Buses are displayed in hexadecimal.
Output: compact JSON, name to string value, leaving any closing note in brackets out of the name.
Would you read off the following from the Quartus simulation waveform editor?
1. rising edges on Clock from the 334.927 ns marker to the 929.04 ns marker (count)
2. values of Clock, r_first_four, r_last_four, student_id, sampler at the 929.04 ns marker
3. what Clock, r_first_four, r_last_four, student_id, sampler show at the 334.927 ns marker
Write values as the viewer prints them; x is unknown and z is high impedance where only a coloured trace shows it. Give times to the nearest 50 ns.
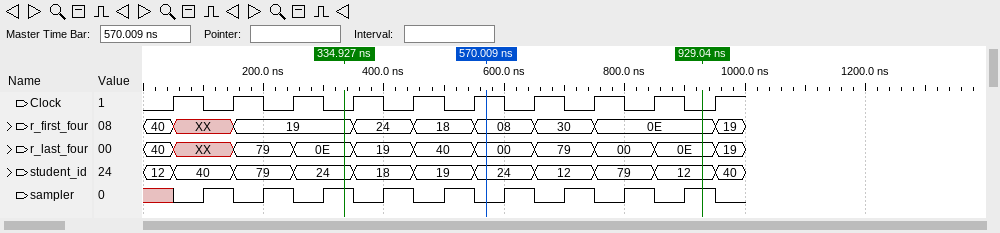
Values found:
{"rising edges on Clock from the 334.927 ns marker to the 929.04 ns marker": "6", "values of Clock, r_first_four, r_last_four, student_id, sampler at the 929.04 ns marker": "Clock=0, r_first_four=0E, r_last_four=0E, student_id=12, sampler=1", "what Clock, r_first_four, r_last_four, student_id, sampler show at the 334.927 ns marker": "Clock=0, r_first_four=19, r_last_four=0E, student_id=24, sampler=1"}
